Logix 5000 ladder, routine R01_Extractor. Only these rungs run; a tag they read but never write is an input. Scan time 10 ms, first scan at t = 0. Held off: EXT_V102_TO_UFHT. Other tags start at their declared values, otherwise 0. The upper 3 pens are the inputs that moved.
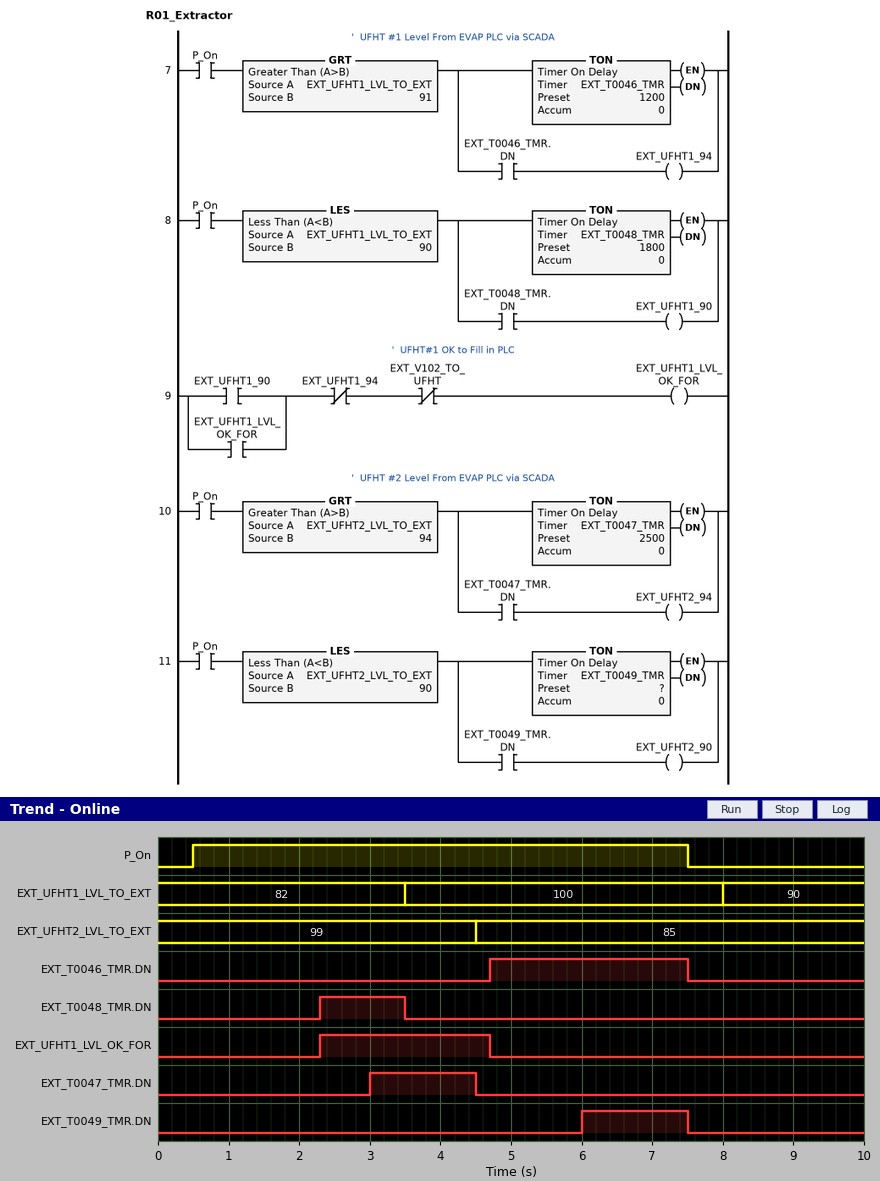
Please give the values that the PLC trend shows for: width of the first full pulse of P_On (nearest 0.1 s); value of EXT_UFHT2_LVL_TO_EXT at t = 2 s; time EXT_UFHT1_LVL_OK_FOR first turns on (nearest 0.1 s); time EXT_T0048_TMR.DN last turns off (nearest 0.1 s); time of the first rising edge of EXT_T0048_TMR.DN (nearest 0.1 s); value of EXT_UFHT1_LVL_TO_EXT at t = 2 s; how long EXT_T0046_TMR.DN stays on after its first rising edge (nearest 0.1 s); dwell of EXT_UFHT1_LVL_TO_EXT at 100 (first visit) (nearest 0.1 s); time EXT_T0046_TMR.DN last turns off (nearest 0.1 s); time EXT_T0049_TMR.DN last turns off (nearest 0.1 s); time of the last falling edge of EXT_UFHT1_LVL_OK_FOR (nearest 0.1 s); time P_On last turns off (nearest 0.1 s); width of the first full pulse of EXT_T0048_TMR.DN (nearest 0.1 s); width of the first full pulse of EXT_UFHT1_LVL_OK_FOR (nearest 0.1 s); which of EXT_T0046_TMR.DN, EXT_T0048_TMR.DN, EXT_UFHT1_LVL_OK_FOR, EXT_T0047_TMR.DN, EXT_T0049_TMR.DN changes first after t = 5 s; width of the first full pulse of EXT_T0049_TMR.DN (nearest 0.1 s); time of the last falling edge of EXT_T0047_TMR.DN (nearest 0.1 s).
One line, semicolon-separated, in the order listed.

7.0 s; 99; 2.3 s; 3.5 s; 2.3 s; 82; 2.8 s; 4.5 s; 7.5 s; 7.5 s; 4.7 s; 7.5 s; 1.2 s; 2.4 s; EXT_T0049_TMR.DN; 1.5 s; 4.5 s
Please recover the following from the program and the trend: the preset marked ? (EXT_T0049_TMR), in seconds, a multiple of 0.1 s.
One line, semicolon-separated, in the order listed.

1.5 s
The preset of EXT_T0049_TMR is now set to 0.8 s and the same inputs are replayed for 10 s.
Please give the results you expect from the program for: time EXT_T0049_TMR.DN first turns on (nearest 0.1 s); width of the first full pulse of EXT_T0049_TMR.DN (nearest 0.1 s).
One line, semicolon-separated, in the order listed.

5.3 s; 2.2 s
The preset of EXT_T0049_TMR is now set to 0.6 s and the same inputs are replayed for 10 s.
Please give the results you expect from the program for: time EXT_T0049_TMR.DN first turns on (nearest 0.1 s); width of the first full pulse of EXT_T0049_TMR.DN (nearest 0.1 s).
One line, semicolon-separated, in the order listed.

5.1 s; 2.4 s
